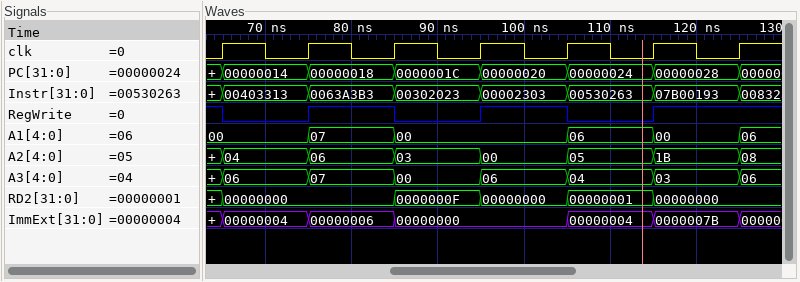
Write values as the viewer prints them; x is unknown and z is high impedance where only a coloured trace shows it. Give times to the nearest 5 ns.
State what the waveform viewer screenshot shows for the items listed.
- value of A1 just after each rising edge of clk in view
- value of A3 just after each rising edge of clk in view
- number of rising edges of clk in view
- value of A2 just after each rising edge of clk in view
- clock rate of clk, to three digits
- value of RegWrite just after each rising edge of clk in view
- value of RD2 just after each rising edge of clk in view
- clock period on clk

00, 07, 00, 00, 06, 00, 06
06, 07, 00, 06, 04, 03, 06
7
04, 06, 03, 00, 05, 1B, 08
100 MHz
0 1 0 1 0 1 1
00000000, 00000000, 0000000F, 00000000, 00000001, 00000000, 00000000
10 ns
